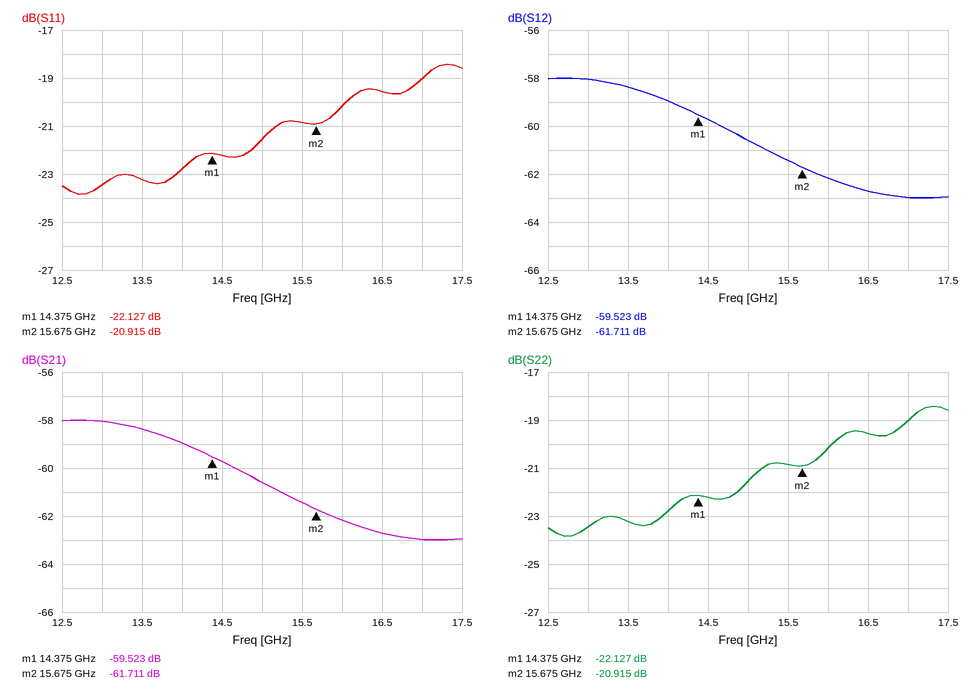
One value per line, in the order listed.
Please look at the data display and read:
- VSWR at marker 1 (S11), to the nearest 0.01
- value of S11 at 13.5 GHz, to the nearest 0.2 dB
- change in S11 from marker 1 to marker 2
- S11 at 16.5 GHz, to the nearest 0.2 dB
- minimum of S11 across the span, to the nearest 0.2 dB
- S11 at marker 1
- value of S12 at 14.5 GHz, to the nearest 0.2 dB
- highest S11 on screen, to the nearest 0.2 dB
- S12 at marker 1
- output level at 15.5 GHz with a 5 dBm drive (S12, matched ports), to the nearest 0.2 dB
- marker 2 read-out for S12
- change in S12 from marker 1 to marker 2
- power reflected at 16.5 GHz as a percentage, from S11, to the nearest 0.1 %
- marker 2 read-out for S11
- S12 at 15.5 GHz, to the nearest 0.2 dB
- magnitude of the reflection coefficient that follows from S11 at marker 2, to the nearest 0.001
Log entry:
1.17
-23.2 dB
1.212 dB
-19.6 dB
-23.8 dB
-22.127 dB
-59.8 dB
-18.4 dB
-59.523 dB
-56.4 dBm
-61.711 dB
-2.188 dB
1.1 %
-20.915 dB
-61.4 dB
0.090
